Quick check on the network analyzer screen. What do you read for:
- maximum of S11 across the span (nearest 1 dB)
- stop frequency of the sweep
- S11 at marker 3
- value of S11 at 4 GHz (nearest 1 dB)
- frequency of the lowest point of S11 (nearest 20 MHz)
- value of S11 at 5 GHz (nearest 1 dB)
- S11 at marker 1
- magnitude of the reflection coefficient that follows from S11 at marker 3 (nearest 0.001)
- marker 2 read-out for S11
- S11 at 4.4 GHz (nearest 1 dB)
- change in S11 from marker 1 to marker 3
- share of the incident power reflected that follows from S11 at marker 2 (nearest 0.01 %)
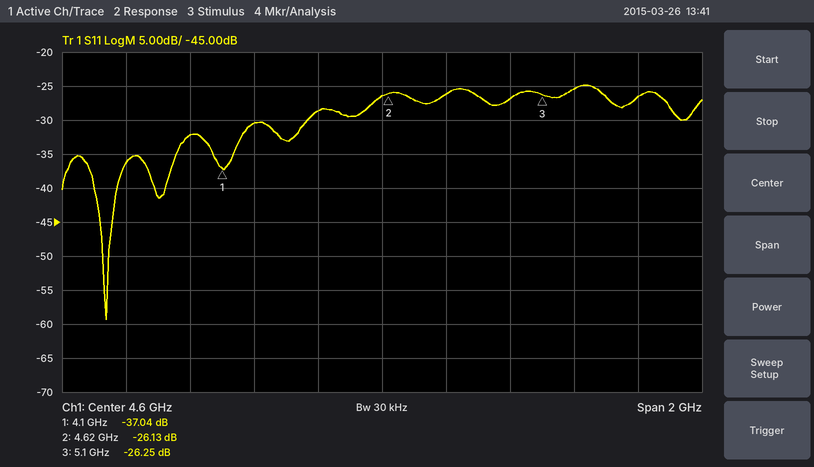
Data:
-25 dB
5.6 GHz
-26.25 dB
-32 dB
3.74 GHz
-27 dB
-37.04 dB
0.049
-26.13 dB
-29 dB
10.79 dB
0.24 %
